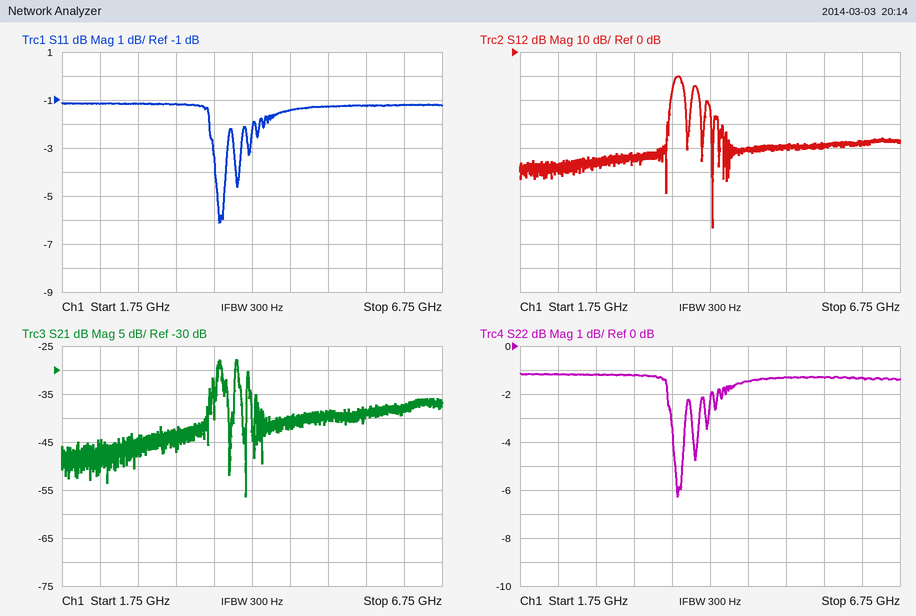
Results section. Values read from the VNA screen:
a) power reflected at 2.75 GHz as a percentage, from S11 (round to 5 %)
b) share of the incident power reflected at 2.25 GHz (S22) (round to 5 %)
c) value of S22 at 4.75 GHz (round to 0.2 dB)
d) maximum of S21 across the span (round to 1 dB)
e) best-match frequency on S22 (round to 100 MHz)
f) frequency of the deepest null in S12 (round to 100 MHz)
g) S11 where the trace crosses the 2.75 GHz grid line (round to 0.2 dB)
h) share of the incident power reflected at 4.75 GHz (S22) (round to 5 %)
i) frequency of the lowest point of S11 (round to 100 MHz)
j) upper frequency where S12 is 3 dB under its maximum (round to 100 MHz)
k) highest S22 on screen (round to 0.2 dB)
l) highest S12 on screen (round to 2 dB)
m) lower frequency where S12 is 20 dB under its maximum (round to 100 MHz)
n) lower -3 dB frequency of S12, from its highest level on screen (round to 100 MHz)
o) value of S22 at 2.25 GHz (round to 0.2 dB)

75 %
75 %
-1.4 dB
-28 dB
3.8 GHz
4.3 GHz
-1.2 dB
70 %
3.8 GHz
3.9 GHz
-1.2 dB
-10 dB
3.7 GHz
3.8 GHz
-1.2 dB
